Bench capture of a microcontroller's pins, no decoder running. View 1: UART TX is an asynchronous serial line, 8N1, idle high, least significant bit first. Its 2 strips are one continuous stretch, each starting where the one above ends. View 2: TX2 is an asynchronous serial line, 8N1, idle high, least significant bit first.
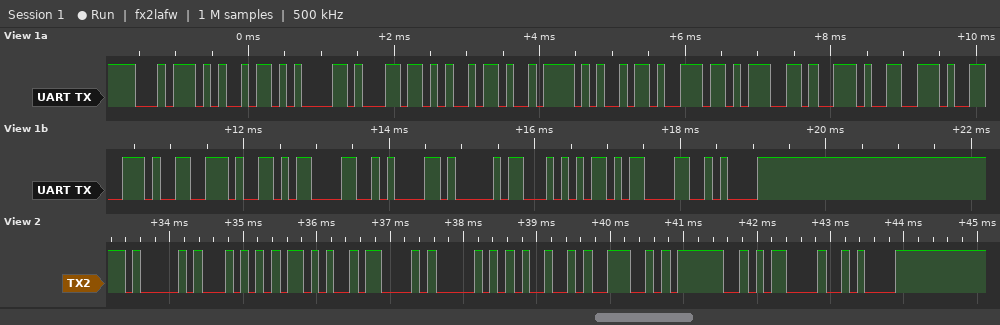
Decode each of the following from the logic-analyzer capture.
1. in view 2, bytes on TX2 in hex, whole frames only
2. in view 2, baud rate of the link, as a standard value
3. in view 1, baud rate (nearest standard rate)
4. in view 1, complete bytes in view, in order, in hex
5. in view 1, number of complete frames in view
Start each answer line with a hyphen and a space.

- 41 54 2B 43 50 49 4E 3F 0D 0A
- 9600 baud
- 9600 baud
- 74 69 61 6C 69 7A 69 6E 67 2E 2E 2E 2E 0D 0A 41 54 0D 0A
- 19
